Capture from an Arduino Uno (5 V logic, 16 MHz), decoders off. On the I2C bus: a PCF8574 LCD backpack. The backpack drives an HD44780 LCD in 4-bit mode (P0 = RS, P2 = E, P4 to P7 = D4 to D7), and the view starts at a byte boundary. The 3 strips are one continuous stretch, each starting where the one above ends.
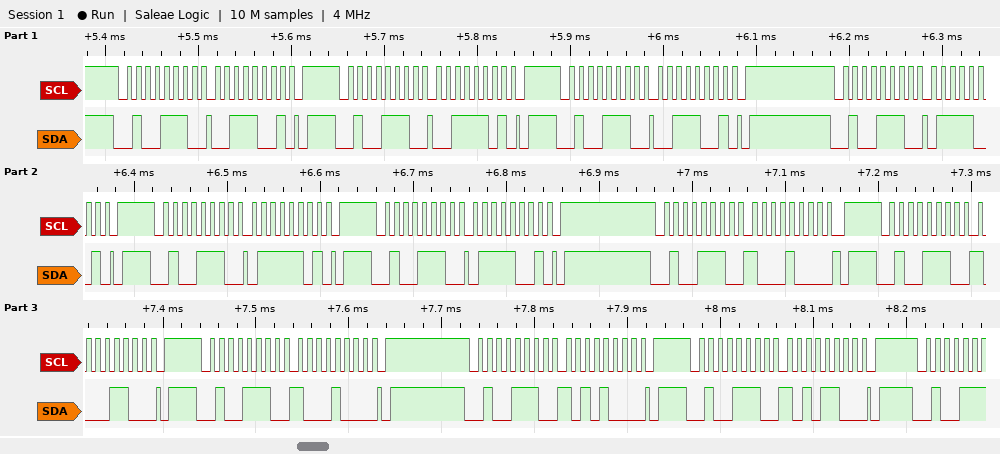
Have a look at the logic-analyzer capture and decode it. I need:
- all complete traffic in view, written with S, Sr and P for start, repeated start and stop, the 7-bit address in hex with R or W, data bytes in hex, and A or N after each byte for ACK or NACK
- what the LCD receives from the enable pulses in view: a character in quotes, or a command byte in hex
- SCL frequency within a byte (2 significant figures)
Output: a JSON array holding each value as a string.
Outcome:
["S 27W A 39 A P S 27W A 3D A P S 27W A 39 A P S 27W A 79 A P S 27W A 7D A P S 27W A 79 A P S 27W A 88 A P S 27W A 8C A P S 27W A 88 A P S 27W A A8 A P S 27W A AC A P", "'7'", "100 kHz"]
